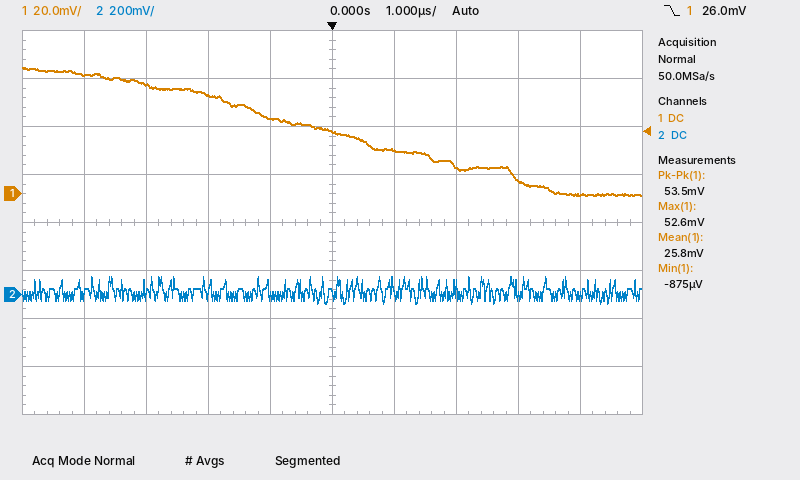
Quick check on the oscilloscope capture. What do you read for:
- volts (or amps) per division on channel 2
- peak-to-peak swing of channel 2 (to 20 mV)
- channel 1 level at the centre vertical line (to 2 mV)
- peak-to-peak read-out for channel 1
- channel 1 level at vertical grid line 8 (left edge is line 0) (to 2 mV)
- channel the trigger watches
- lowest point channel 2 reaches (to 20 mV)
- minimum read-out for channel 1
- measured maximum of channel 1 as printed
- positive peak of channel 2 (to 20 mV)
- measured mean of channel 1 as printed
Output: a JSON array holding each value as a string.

["200 mV", "120 mV", "26 mV", "53.5 mV", "6 mV", "channel 1", "-40 mV", "-875 µV", "52.6 mV", "80 mV", "25.8 mV"]
